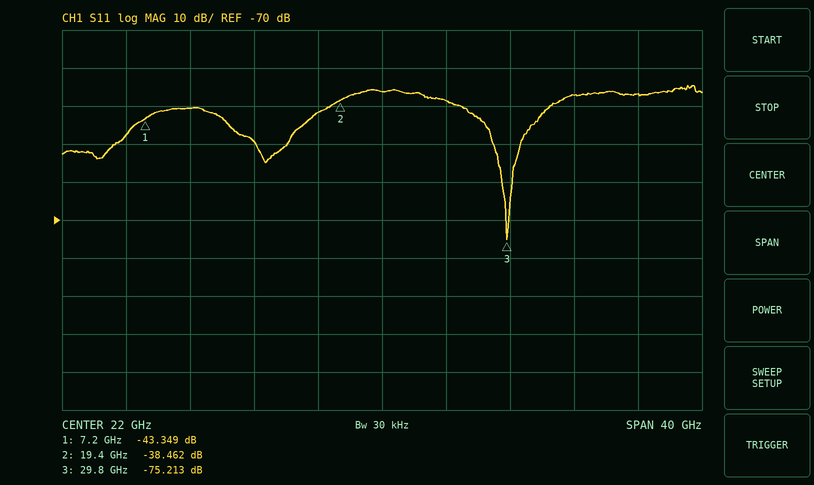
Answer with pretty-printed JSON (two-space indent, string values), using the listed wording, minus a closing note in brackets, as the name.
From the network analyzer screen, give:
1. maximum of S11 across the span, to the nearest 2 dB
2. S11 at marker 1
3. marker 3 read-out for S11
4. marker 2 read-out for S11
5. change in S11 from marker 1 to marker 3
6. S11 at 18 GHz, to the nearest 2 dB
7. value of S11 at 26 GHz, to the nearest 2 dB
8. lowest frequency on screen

{
  "maximum of S11 across the span, to the nearest 2 dB": "-34 dB",
  "S11 at marker 1": "-43.349 dB",
  "marker 3 read-out for S11": "-75.213 dB",
  "marker 2 read-out for S11": "-38.462 dB",
  "change in S11 from marker 1 to marker 3": "-31.864 dB",
  "S11 at 18 GHz, to the nearest 2 dB": "-42 dB",
  "value of S11 at 26 GHz, to the nearest 2 dB": "-38 dB",
  "lowest frequency on screen": "2 GHz"
}
